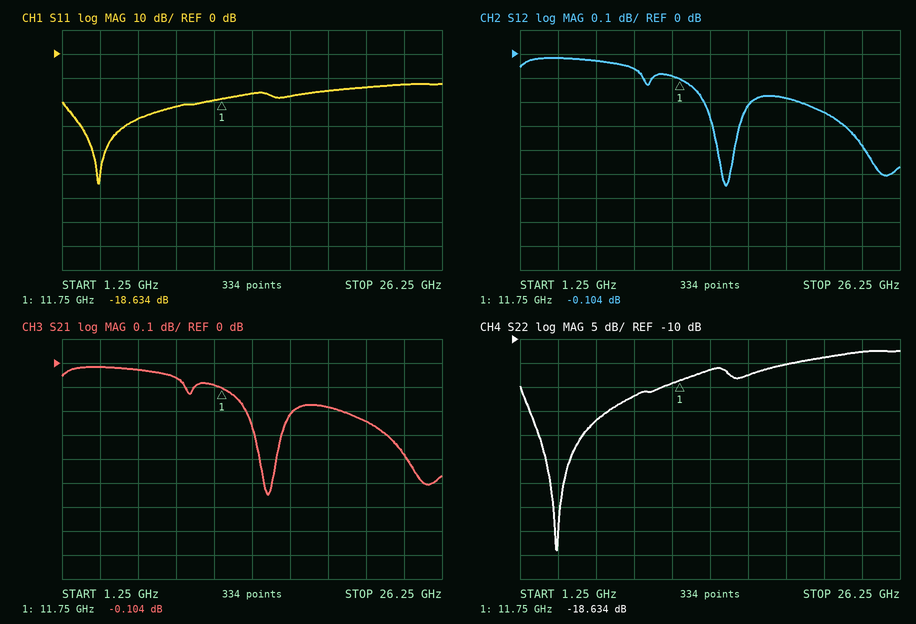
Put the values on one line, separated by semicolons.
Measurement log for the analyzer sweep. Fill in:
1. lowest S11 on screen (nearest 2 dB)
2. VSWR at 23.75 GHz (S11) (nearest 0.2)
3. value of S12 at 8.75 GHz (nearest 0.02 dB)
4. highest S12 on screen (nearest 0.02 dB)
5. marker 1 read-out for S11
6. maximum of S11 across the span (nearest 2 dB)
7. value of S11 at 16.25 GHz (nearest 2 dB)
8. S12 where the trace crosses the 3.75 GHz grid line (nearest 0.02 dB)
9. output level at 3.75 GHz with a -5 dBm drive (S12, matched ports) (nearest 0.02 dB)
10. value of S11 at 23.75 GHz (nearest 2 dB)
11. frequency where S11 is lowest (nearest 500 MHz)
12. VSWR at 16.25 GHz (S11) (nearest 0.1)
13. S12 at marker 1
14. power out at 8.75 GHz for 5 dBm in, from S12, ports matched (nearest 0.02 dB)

-54 dB; 1.6; -0.06 dB; -0.02 dB; -18.634 dB; -12 dB; -18 dB; -0.02 dB; -5.02 dBm; -12 dB; 3.5 GHz; 1.3; -0.104 dB; 4.94 dBm
